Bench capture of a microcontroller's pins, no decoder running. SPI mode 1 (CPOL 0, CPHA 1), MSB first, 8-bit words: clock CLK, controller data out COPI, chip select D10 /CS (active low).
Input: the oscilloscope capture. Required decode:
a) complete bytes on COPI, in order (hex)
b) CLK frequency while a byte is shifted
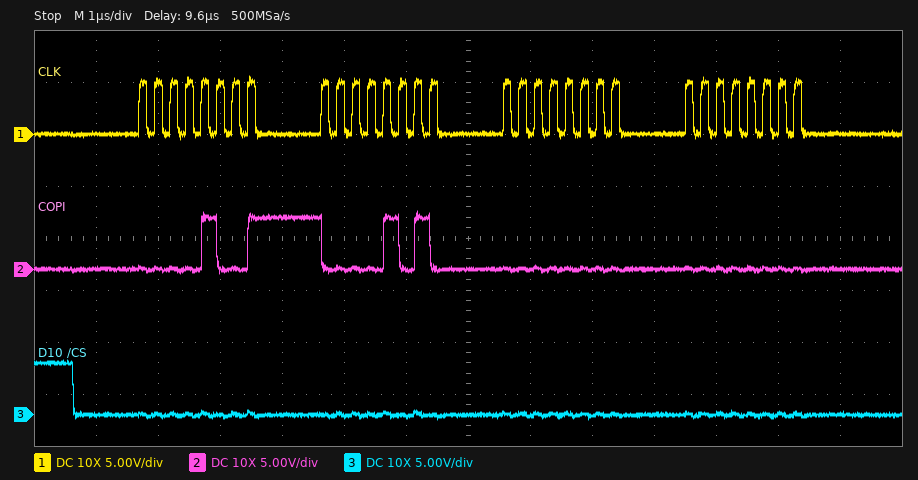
09 0A 00 00
4 MHz
